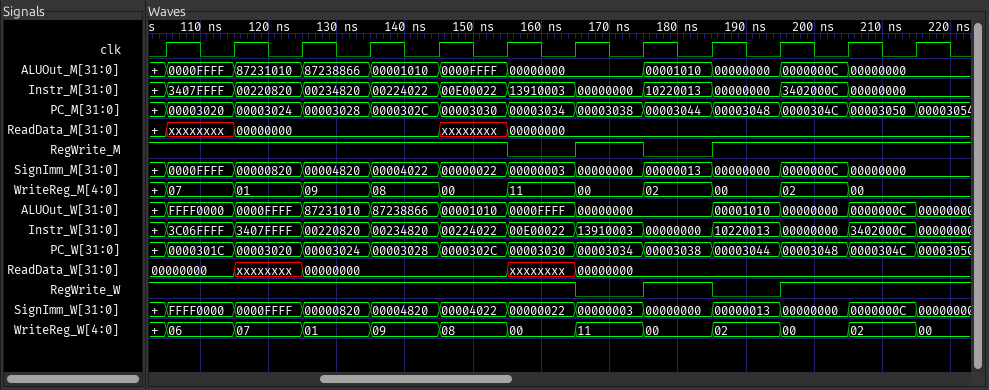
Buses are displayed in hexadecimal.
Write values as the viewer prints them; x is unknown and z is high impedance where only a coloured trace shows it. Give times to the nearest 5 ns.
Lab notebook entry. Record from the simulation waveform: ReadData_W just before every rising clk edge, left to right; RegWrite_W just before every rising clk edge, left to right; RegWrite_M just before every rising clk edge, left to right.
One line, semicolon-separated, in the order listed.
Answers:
00000000, 00000000, xxxxxxxx, 00000000, 00000000, 00000000, xxxxxxxx, 00000000, 00000000, 00000000, 00000000, 00000000; 1 1 1 1 1 1 1 0 1 0 1 1; 1 1 1 1 1 1 0 1 0 1 1 1
